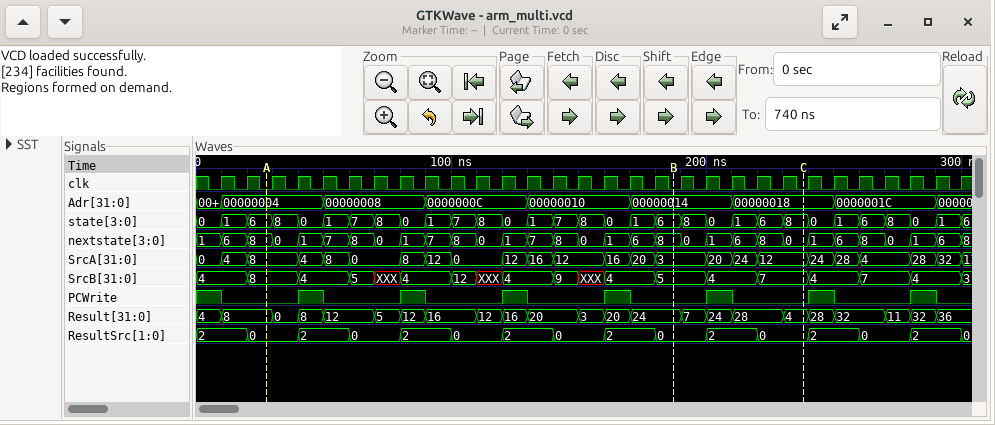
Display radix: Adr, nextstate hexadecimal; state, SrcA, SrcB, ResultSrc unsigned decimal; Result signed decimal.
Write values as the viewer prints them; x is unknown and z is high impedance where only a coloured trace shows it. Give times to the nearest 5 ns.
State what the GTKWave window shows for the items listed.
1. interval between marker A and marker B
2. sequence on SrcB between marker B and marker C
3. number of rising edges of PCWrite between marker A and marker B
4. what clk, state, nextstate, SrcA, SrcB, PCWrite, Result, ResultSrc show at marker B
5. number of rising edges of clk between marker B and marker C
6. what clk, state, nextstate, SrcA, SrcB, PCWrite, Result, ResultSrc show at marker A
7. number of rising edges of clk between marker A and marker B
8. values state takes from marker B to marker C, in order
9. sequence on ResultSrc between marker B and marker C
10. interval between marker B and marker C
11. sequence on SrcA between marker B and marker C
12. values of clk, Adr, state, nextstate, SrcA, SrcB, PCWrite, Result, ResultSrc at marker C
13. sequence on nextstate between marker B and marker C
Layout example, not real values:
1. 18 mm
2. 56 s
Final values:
1. 160 ns
2. 5, 4, 7
3. 4
4. clk=0, state=6, nextstate=8, SrcA=3, SrcB=5, PCWrite=0, Result=24, ResultSrc=0
5. 5
6. clk=0, state=6, nextstate=8, SrcA=8, SrcB=8, PCWrite=0, Result=8, ResultSrc=0
7. 16
8. 6, 8, 0, 1, 6, 8
9. 0, 2, 0
10. 50 ns
11. 3, 20, 24, 12
12. clk=0, Adr=00000018, state=8, nextstate=0, SrcA=12, SrcB=7, PCWrite=0, Result=4, ResultSrc=0
13. 8, 0, 1, 6, 8, 0
